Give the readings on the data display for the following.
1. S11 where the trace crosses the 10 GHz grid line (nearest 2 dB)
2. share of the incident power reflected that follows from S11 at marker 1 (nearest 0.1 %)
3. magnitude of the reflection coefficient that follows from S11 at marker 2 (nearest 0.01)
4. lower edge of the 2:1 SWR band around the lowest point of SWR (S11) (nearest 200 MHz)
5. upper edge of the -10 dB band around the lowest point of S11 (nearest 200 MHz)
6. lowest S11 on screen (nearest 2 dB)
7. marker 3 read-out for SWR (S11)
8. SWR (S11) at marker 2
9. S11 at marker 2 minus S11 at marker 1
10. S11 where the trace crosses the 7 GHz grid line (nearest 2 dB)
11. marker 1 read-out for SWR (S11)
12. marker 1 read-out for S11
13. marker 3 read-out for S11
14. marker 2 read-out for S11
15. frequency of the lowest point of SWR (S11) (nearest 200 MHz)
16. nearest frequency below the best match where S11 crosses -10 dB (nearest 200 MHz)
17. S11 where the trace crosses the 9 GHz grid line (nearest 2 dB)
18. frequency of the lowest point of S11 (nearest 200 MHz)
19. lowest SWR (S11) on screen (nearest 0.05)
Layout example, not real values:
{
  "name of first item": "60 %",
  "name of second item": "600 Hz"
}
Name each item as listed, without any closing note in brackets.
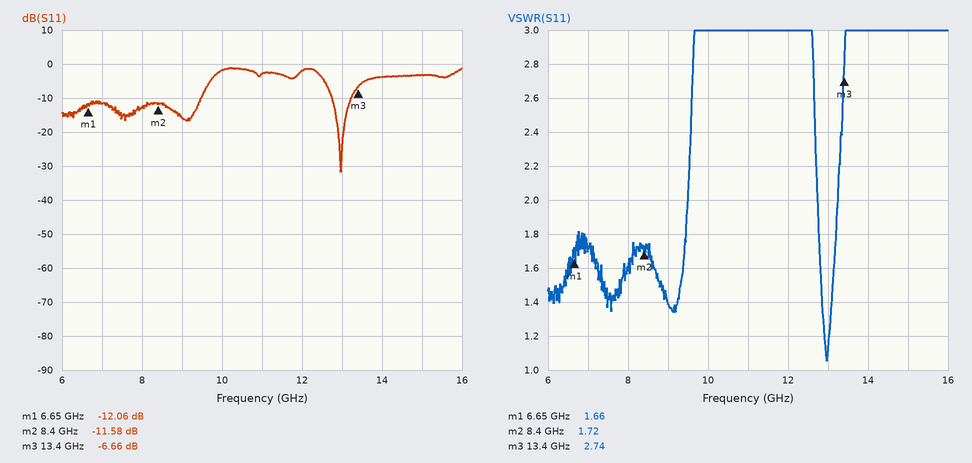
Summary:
{
  "S11 where the trace crosses the 10 GHz grid line": "-2 dB",
  "share of the incident power reflected that follows from S11 at marker 1": "6.2 %",
  "magnitude of the reflection coefficient that follows from S11 at marker 2": "0.26",
  "lower edge of the 2:1 SWR band around the lowest point of SWR (S11)": "12.8 GHz",
  "upper edge of the -10 dB band around the lowest point of S11": "13.2 GHz",
  "lowest S11 on screen": "-32 dB",
  "marker 3 read-out for SWR": "2.74",
  "SWR (S11) at marker 2": "1.72",
  "S11 at marker 2 minus S11 at marker 1": "0.48 dB",
  "S11 where the trace crosses the 7 GHz grid line": "-12 dB",
  "marker 1 read-out for SWR": "1.66",
  "marker 1 read-out for S11": "-12.06 dB",
  "marker 3 read-out for S11": "-6.66 dB",
  "marker 2 read-out for S11": "-11.58 dB",
  "frequency of the lowest point of SWR (S11)": "13.0 GHz",
  "nearest frequency below the best match where S11 crosses -10 dB": "12.8 GHz",
  "S11 where the trace crosses the 9 GHz grid line": "-16 dB",
  "frequency of the lowest point of S11": "13.0 GHz",
  "lowest SWR (S11) on screen": "1.05"
}
